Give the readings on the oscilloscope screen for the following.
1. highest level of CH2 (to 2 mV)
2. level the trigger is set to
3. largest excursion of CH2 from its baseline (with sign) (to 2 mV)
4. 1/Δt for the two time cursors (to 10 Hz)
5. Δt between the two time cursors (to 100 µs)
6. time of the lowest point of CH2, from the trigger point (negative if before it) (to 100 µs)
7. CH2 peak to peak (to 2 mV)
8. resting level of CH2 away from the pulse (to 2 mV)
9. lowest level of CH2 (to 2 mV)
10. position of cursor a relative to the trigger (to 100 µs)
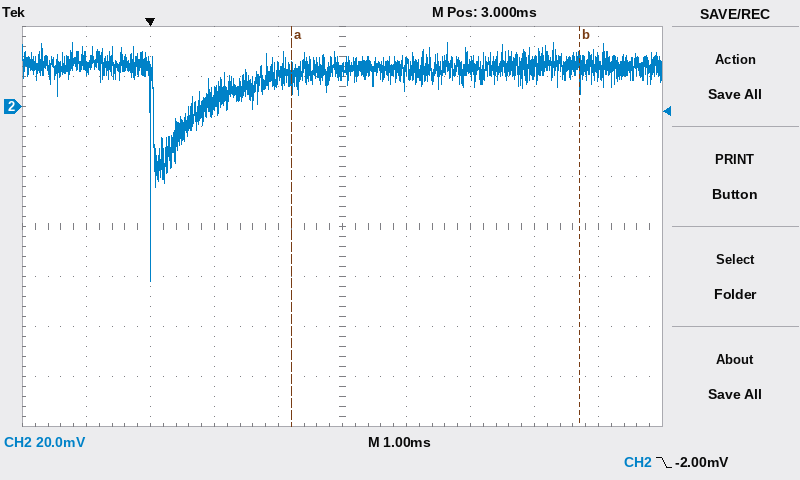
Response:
26 mV
-2.00 mV
-86 mV
220 Hz
4.5 ms
0.0 ms
96 mV
16 mV
-70 mV
+2.2 ms
